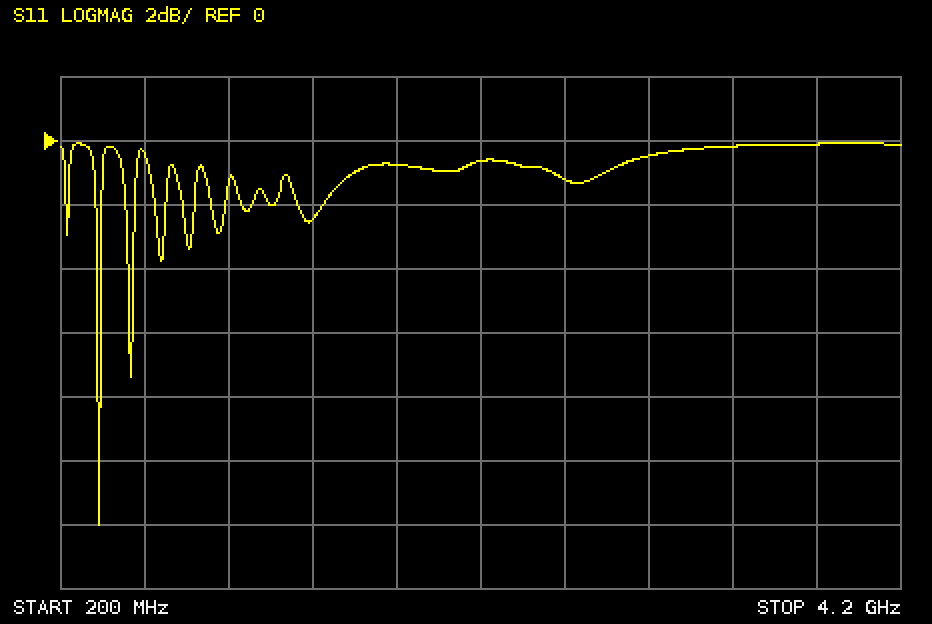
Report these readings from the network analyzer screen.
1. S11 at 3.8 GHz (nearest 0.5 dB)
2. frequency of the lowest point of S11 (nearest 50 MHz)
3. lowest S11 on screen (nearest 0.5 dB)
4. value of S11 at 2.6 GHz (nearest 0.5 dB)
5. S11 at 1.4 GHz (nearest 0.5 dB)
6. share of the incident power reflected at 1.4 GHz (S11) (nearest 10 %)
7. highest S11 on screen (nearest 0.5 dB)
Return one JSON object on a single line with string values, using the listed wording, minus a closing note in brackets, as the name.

{"S11 at 3.8 GHz": "0.0 dB", "frequency of the lowest point of S11": "400 MHz", "lowest S11 on screen": "-12.0 dB", "value of S11 at 2.6 GHz": "-1.0 dB", "S11 at 1.4 GHz": "-2.5 dB", "share of the incident power reflected at 1.4 GHz (S11)": "60 %", "highest S11 on screen": "0.0 dB"}
